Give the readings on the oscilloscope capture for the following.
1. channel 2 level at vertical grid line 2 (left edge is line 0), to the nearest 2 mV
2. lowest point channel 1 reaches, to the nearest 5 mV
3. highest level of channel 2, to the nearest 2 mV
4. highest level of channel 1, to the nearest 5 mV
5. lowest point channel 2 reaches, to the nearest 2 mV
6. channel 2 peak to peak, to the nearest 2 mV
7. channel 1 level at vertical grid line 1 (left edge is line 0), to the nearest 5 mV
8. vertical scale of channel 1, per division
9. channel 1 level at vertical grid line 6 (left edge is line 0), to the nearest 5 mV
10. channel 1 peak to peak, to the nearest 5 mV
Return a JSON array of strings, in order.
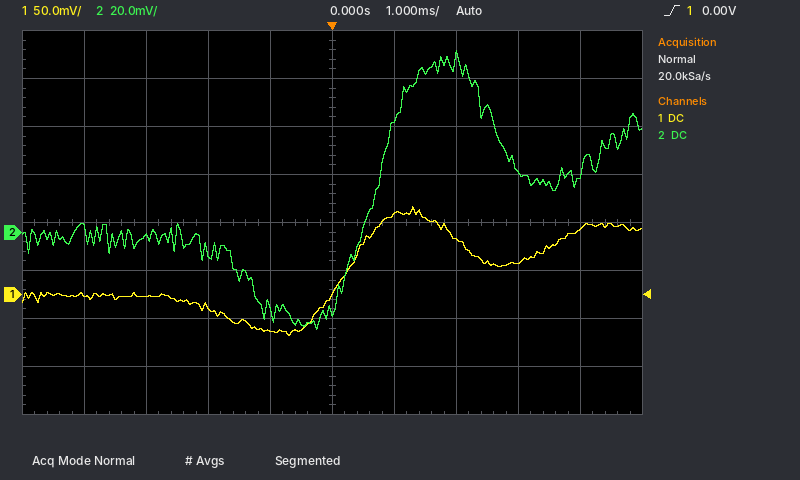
["-2 mV", "-45 mV", "76 mV", "90 mV", "-40 mV", "116 mV", "0 mV", "50 mV", "85 mV", "135 mV"]
